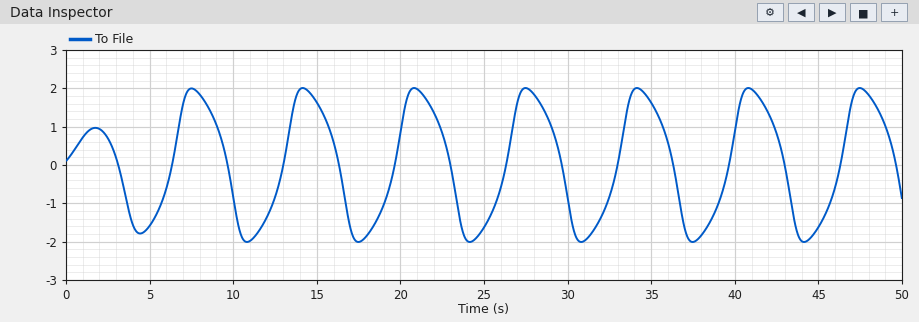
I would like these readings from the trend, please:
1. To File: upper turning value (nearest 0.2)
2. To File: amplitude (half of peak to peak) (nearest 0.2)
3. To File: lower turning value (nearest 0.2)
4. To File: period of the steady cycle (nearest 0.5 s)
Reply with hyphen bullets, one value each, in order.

- 2.0
- 2.0
- -2.0
- 6.5 s
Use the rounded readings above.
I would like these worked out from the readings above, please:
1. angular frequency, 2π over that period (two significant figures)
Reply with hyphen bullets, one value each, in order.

- 0.97 rad/s
